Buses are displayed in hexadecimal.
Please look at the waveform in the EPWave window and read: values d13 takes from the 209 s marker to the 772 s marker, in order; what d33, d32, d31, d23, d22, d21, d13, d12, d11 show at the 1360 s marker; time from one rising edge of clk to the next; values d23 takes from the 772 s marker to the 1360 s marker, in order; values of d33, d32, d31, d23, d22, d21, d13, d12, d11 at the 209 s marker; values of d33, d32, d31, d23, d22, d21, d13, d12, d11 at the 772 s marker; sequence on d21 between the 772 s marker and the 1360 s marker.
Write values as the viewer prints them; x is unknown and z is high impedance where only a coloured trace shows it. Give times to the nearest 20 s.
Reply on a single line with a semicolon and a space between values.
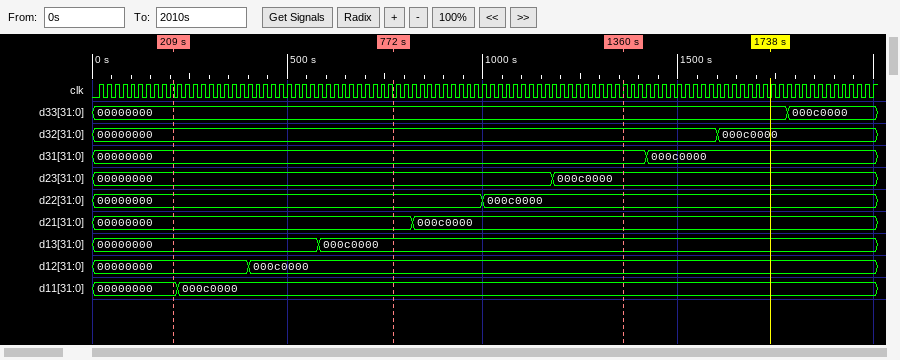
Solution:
00000000, 000c0000; d33=00000000, d32=00000000, d31=00000000, d23=000c0000, d22=000c0000, d21=000c0000, d13=000c0000, d12=000c0000, d11=000c0000; 20 s; 00000000, 000c0000; d33=00000000, d32=00000000, d31=00000000, d23=00000000, d22=00000000, d21=00000000, d13=00000000, d12=00000000, d11=00000000; d33=00000000, d32=00000000, d31=00000000, d23=00000000, d22=00000000, d21=00000000, d13=000c0000, d12=000c0000, d11=000c0000; 00000000, 000c0000
